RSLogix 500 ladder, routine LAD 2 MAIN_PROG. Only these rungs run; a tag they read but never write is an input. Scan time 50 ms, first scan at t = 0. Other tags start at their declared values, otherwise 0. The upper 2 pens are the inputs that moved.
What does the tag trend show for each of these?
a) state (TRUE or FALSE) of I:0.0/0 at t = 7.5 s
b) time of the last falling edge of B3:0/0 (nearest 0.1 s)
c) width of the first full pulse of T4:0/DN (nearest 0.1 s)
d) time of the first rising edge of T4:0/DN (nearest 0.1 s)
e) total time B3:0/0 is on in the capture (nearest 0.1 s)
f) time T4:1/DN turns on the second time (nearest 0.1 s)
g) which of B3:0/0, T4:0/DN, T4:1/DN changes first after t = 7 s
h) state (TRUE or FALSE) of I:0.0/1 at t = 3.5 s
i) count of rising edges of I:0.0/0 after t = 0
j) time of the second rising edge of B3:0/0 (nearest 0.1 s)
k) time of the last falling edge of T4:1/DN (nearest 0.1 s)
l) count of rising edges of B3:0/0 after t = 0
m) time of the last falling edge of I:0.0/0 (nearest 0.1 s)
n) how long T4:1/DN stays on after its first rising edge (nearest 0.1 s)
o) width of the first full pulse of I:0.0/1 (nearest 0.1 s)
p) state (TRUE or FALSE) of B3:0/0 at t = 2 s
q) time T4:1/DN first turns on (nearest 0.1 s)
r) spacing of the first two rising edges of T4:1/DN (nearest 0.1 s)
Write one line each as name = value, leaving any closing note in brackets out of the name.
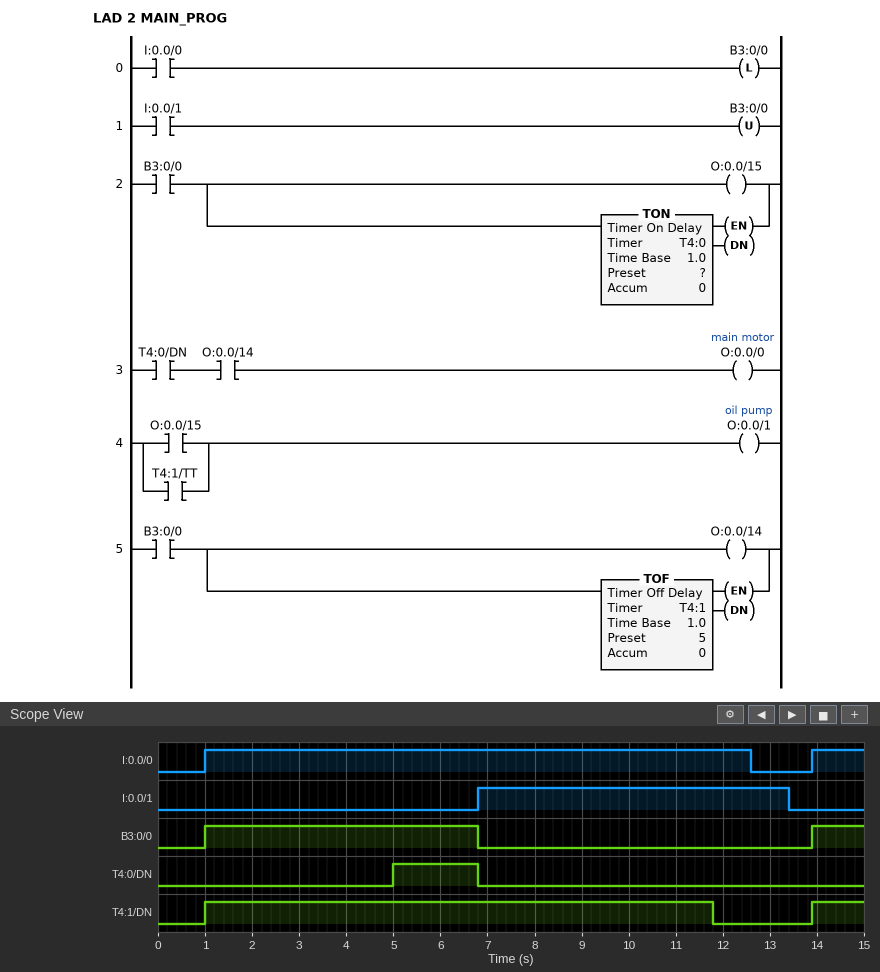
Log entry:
state (TRUE or FALSE) of I:0.0/0 at t = 7.5 s = TRUE
time of the last falling edge of B3:0/0 = 6.8 s
width of the first full pulse of T4:0/DN = 1.8 s
time of the first rising edge of T4:0/DN = 5.0 s
total time B3:0/0 is on in the capture = 6.9 s
time T4:1/DN turns on the second time = 13.9 s
which of B3:0/0, T4:0/DN, T4:1/DN changes first after t = 7 s = T4:1/DN
state (TRUE or FALSE) of I:0.0/1 at t = 3.5 s = FALSE
count of rising edges of I:0.0/0 after t = 0 = 2
time of the second rising edge of B3:0/0 = 13.9 s
time of the last falling edge of T4:1/DN = 11.8 s
count of rising edges of B3:0/0 after t = 0 = 2
time of the last falling edge of I:0.0/0 = 12.6 s
how long T4:1/DN stays on after its first rising edge = 10.8 s
width of the first full pulse of I:0.0/1 = 6.6 s
state (TRUE or FALSE) of B3:0/0 at t = 2 s = TRUE
time T4:1/DN first turns on = 1.0 s
spacing of the first two rising edges of T4:1/DN = 12.9 s
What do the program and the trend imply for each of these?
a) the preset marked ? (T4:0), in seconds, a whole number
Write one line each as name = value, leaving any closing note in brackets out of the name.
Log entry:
the preset marked ? (T4:0), in seconds, a whole number = 4 s
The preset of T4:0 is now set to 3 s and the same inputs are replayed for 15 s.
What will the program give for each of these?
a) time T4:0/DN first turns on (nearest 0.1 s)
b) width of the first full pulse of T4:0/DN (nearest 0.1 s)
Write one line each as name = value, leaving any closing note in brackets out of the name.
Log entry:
time T4:0/DN first turns on = 4.0 s
width of the first full pulse of T4:0/DN = 2.8 s
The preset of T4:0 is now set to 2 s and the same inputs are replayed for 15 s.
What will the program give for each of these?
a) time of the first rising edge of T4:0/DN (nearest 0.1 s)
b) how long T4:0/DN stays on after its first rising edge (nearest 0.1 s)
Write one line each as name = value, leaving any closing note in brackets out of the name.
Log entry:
time of the first rising edge of T4:0/DN = 3.0 s
how long T4:0/DN stays on after its first rising edge = 3.8 s
